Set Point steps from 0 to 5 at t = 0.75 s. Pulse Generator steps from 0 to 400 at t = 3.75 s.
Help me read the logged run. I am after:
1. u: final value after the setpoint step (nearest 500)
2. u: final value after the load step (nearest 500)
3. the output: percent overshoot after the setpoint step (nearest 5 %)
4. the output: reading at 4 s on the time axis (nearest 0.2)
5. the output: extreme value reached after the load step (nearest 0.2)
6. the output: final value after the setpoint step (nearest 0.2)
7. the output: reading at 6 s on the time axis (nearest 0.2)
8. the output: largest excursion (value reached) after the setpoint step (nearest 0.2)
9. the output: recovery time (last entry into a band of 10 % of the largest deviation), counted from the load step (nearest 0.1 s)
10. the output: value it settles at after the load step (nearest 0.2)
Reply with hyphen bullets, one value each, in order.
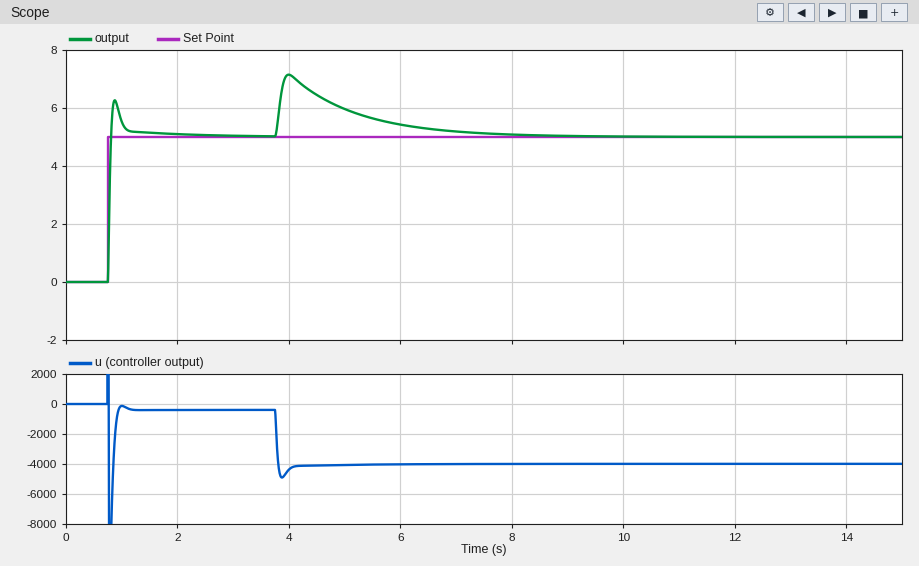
- -500
- -4000
- 25 %
- 7.2
- 7.2
- 5.0
- 5.4
- 6.2
- 3.1 s
- 5.0
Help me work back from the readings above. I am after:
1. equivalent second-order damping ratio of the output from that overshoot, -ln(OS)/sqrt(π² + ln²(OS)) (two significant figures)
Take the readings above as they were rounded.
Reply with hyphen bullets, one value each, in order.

- 0.40
